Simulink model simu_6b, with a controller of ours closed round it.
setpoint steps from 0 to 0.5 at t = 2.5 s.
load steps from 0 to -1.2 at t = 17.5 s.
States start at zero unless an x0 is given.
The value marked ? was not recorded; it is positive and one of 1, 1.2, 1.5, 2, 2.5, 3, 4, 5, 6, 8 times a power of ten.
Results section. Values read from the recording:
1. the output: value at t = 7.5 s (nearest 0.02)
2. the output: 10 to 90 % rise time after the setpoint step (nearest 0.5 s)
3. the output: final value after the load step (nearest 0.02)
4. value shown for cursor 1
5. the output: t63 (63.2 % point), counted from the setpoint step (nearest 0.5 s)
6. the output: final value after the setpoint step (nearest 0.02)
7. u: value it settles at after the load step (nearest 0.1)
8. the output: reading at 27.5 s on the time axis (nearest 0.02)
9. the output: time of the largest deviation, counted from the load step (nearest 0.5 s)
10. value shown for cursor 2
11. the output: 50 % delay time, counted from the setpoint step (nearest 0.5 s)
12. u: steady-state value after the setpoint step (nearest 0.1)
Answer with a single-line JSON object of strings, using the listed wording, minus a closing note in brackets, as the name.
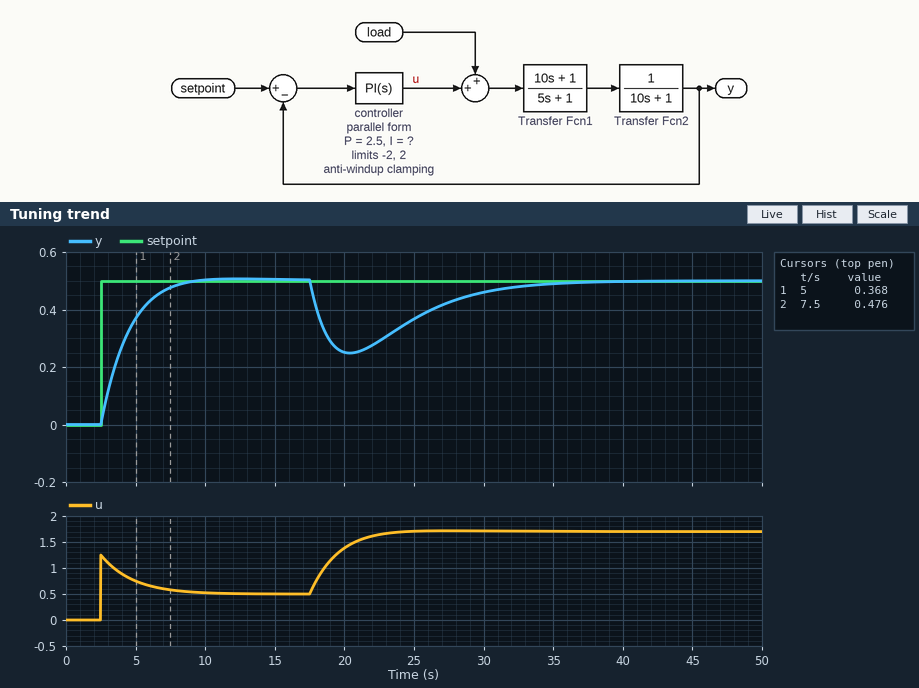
{"the output: value at t = 7.5 s": "0.48", "the output: 10 to 90 % rise time after the setpoint step": "4.0 s", "the output: final value after the load step": "0.50", "value shown for cursor 1": "0.368", "the output: t63 (63.2 % point), counted from the setpoint step": "2.0 s", "the output: final value after the setpoint step": "0.50", "u: value it settles at after the load step": "1.7", "the output: reading at 27.5 s on the time axis": "0.42", "the output: time of the largest deviation, counted from the load step": "3.0 s", "value shown for cursor 2": "0.476", "the output: 50 % delay time, counted from the setpoint step": "1.5 s", "u: steady-state value after the setpoint step": "0.5"}
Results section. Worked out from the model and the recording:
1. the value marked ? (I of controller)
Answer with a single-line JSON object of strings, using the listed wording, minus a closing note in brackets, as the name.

{"the value marked ?": "0.6"}
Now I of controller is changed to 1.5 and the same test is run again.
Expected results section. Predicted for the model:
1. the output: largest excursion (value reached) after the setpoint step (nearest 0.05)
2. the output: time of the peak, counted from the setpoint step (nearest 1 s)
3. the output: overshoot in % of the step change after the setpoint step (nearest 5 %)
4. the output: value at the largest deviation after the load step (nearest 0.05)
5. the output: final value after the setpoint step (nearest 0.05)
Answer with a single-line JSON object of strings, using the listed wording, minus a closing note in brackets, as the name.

{"the output: largest excursion (value reached) after the setpoint step": "0.55", "the output: time of the peak, counted from the setpoint step": "5 s", "the output: overshoot in % of the step change after the setpoint step": "15 %", "the output: value at the largest deviation after the load step": "0.30", "the output: final value after the setpoint step": "0.50"}
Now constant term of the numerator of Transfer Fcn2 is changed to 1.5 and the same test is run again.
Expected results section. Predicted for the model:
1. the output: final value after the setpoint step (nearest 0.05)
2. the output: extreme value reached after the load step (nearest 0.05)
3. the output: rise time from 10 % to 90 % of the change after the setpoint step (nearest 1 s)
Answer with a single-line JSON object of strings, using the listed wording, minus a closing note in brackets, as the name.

{"the output: final value after the setpoint step": "0.50", "the output: extreme value reached after the load step": "0.20", "the output: rise time from 10 % to 90 % of the change after the setpoint step": "3 s"}
